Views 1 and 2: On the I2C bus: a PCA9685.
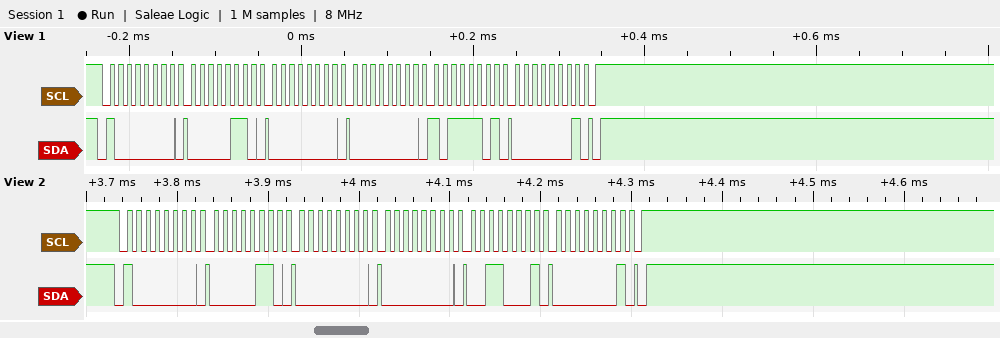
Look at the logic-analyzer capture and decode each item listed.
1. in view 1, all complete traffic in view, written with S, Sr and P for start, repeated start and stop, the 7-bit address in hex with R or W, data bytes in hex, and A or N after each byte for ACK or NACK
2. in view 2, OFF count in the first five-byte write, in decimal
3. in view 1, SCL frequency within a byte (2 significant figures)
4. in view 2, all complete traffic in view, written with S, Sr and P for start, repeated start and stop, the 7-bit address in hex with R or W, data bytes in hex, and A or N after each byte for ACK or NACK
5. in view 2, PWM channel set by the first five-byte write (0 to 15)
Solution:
S 40W A 06 A 00 A 00 A BD A 01 A P
305
100 kHz
S 40W A 06 A 00 A 00 A 31 A 01 A P
0
